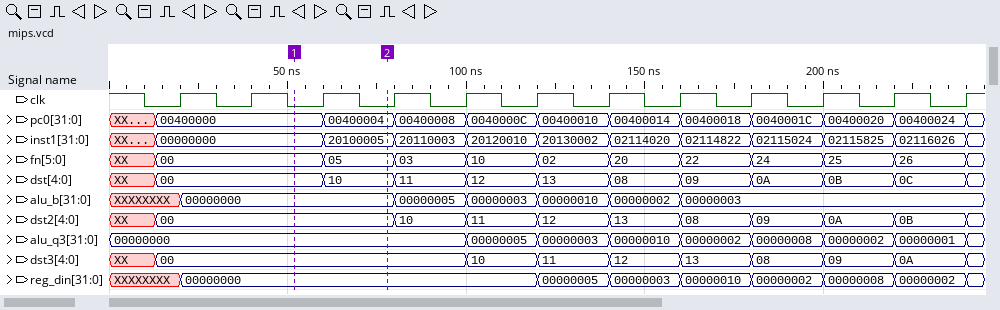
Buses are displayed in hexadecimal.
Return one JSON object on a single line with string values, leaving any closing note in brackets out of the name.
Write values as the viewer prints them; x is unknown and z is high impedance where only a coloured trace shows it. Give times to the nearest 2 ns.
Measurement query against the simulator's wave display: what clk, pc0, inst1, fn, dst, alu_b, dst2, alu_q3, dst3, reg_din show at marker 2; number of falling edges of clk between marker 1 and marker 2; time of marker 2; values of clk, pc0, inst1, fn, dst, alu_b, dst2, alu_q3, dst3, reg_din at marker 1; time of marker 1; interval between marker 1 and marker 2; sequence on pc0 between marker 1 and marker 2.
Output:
{"what clk, pc0, inst1, fn, dst, alu_b, dst2, alu_q3, dst3, reg_din show at marker 2": "clk=0, pc0=00400004, inst1=20100005, fn=05, dst=10, alu_b=00000000, dst2=00, alu_q3=00000000, dst3=00, reg_din=00000000", "number of falling edges of clk between marker 1 and marker 2": "1", "time of marker 2": "78 ns", "values of clk, pc0, inst1, fn, dst, alu_b, dst2, alu_q3, dst3, reg_din at marker 1": "clk=0, pc0=00400000, inst1=00000000, fn=00, dst=00, alu_b=00000000, dst2=00, alu_q3=00000000, dst3=00, reg_din=00000000", "time of marker 1": "52 ns", "interval between marker 1 and marker 2": "26 ns", "sequence on pc0 between marker 1 and marker 2": "00400000, 00400004"}
